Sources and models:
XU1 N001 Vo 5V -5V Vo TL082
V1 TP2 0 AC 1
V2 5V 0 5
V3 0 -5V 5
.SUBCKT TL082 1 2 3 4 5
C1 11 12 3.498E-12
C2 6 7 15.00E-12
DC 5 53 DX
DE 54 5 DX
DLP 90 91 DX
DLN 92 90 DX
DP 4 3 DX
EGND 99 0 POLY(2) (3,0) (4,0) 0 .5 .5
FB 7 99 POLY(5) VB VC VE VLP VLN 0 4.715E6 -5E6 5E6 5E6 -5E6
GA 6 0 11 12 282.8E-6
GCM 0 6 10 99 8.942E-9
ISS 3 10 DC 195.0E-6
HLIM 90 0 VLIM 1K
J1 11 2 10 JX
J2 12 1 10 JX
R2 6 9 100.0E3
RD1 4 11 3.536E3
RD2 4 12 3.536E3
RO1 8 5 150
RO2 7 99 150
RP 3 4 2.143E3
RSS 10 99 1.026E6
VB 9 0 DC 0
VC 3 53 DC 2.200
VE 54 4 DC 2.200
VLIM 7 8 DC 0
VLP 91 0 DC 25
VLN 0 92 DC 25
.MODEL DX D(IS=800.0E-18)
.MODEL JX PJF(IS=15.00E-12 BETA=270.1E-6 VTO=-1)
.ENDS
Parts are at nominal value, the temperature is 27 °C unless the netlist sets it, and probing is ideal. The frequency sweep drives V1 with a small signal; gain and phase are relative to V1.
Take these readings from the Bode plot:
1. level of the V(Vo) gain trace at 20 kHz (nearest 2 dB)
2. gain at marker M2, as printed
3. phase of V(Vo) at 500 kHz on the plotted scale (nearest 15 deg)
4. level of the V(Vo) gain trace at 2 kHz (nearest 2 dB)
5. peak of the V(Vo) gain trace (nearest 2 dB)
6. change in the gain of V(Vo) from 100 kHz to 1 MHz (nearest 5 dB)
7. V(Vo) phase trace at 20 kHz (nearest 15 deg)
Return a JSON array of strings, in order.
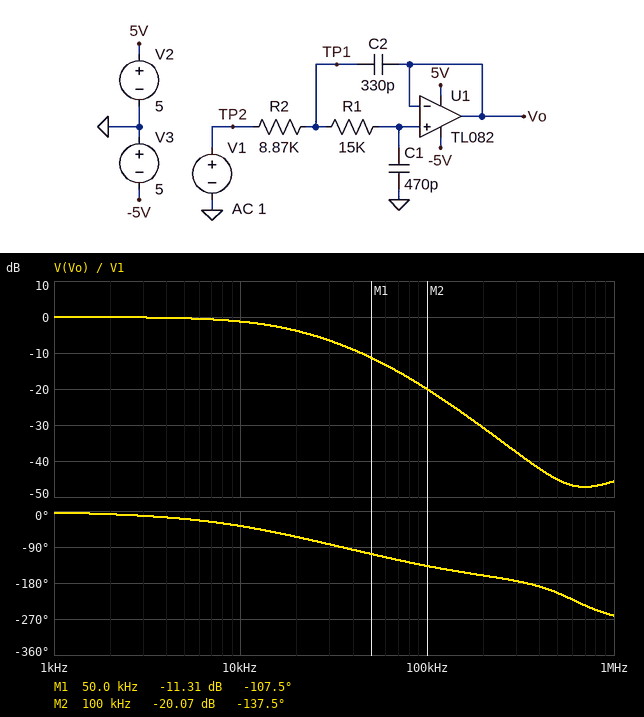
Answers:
["-4 dB", "-20.07 dB", "-210 deg", "0 dB", "0 dB", "-25 dB", "-60 deg"]
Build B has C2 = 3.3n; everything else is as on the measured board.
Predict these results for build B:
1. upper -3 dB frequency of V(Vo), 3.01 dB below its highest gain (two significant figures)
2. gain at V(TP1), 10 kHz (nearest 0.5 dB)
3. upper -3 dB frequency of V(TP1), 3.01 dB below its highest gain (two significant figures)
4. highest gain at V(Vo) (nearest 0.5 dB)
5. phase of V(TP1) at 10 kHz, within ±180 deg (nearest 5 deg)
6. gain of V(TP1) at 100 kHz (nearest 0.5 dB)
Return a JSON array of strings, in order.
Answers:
["13 kHz", "3.5 dB", "14 kHz", "3.0 dB", "-50 deg", "-25.0 dB"]
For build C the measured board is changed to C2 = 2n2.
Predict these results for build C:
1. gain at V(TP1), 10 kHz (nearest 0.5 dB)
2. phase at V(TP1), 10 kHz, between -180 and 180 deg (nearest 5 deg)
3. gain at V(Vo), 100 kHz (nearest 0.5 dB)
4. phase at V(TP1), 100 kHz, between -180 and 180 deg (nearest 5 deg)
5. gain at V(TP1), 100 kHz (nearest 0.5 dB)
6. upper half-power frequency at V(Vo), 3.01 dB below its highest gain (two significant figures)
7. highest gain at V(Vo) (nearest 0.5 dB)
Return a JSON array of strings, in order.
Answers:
["2.5 dB", "-35 deg", "-34.5 dB", "-95 deg", "-21.5 dB", "16 kHz", "1.5 dB"]
